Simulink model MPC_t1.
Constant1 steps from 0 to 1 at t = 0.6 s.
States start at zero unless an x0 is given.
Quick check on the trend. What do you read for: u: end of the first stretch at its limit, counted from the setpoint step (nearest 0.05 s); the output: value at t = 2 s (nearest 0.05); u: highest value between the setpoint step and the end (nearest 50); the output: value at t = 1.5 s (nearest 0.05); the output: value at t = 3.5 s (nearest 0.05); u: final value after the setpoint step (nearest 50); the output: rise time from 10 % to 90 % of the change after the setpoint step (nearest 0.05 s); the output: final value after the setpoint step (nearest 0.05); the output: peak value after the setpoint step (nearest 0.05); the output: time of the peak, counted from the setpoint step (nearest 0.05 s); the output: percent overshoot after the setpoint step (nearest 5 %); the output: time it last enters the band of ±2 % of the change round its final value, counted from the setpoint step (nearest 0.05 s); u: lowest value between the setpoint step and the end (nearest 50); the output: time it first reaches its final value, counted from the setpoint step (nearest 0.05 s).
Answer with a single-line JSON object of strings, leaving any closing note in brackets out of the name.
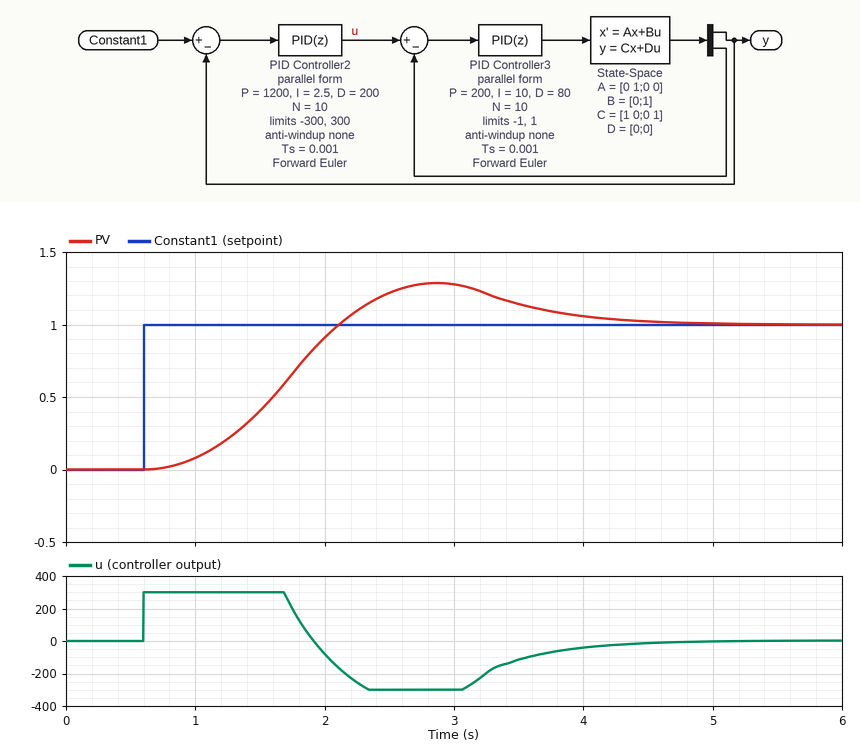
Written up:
{"u: end of the first stretch at its limit, counted from the setpoint step": "1.10 s", "the output: value at t = 2 s": "0.90", "u: highest value between the setpoint step and the end": "300", "the output: value at t = 1.5 s": "0.40", "the output: value at t = 3.5 s": "1.15", "u: final value after the setpoint step": "0", "the output: rise time from 10 % to 90 % of the change after the setpoint step": "0.95 s", "the output: final value after the setpoint step": "1.00", "the output: peak value after the setpoint step": "1.30", "the output: time of the peak, counted from the setpoint step": "2.25 s", "the output: percent overshoot after the setpoint step": "30 %", "the output: time it last enters the band of ±2 % of the change round its final value, counted from the setpoint step": "3.90 s", "u: lowest value between the setpoint step and the end": "-300", "the output: time it first reaches its final value, counted from the setpoint step": "1.50 s"}
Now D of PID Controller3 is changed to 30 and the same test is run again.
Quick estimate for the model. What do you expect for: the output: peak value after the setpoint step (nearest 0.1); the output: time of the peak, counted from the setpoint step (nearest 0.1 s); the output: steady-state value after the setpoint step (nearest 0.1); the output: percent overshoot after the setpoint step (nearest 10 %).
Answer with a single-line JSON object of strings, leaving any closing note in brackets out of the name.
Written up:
{"the output: peak value after the setpoint step": "1.4", "the output: time of the peak, counted from the setpoint step": "2.4 s", "the output: steady-state value after the setpoint step": "1.0", "the output: percent overshoot after the setpoint step": "40 %"}
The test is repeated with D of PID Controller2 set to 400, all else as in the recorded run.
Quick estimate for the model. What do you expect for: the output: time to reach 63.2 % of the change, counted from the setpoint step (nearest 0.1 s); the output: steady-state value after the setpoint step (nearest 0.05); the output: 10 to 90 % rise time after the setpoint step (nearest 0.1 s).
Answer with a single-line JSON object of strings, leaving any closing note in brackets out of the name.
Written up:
{"the output: time to reach 63.2 % of the change, counted from the setpoint step": "1.1 s", "the output: steady-state value after the setpoint step": "1.00", "the output: 10 to 90 % rise time after the setpoint step": "1.1 s"}
